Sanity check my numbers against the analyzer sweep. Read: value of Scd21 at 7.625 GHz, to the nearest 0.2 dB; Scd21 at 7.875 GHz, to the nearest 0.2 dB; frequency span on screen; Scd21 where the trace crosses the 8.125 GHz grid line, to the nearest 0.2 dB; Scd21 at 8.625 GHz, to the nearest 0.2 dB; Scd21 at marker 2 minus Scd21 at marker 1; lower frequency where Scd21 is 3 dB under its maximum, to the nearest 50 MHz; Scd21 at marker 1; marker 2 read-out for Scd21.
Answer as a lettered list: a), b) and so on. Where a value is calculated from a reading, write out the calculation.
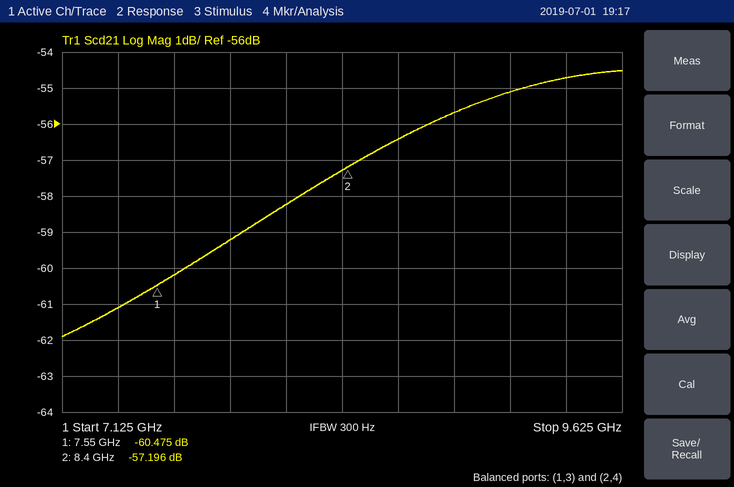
a) -60.2 dB
b) -59.2 dB
c) 2.5 GHz
d) -58.2 dB
e) -56.4 dB
f) -57.196 − (-60.475) = 3.279 dB
g) 8.30 GHz
h) -60.475 dB
i) -57.196 dB
